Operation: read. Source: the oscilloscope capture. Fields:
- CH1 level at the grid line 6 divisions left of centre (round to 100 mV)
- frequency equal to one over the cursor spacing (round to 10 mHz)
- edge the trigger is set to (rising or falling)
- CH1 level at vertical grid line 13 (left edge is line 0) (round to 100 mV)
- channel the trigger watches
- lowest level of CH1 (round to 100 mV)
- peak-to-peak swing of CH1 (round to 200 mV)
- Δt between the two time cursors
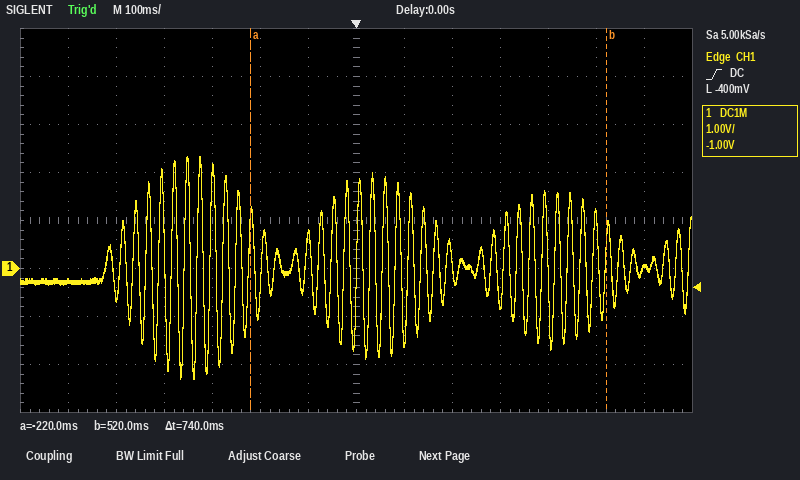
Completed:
-300 mV
1.35 Hz
rising
0.0 V
CH1
-2.3 V
4.6 V
740 ms
